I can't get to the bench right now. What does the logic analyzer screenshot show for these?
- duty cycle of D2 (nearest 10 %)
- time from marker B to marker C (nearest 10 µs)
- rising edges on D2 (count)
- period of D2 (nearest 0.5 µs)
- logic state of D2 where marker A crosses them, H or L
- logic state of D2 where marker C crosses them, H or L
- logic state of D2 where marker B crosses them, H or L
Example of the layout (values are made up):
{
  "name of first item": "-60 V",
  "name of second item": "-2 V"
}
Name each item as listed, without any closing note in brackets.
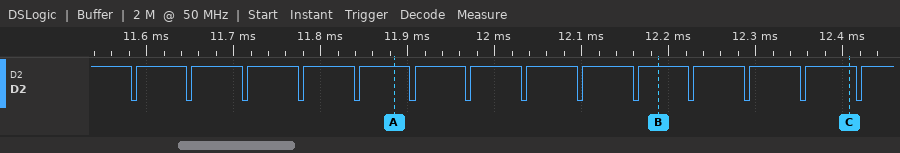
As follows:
{
  "duty cycle of D2": "90 %",
  "time from marker B to marker C": "220 µs",
  "rising edges on D2": "14",
  "period of D2": "64 µs",
  "logic state of D2 where marker A crosses them, H or L": "D2=H",
  "logic state of D2 where marker C crosses them, H or L": "D2=H",
  "logic state of D2 where marker B crosses them, H or L": "D2=H"
}
